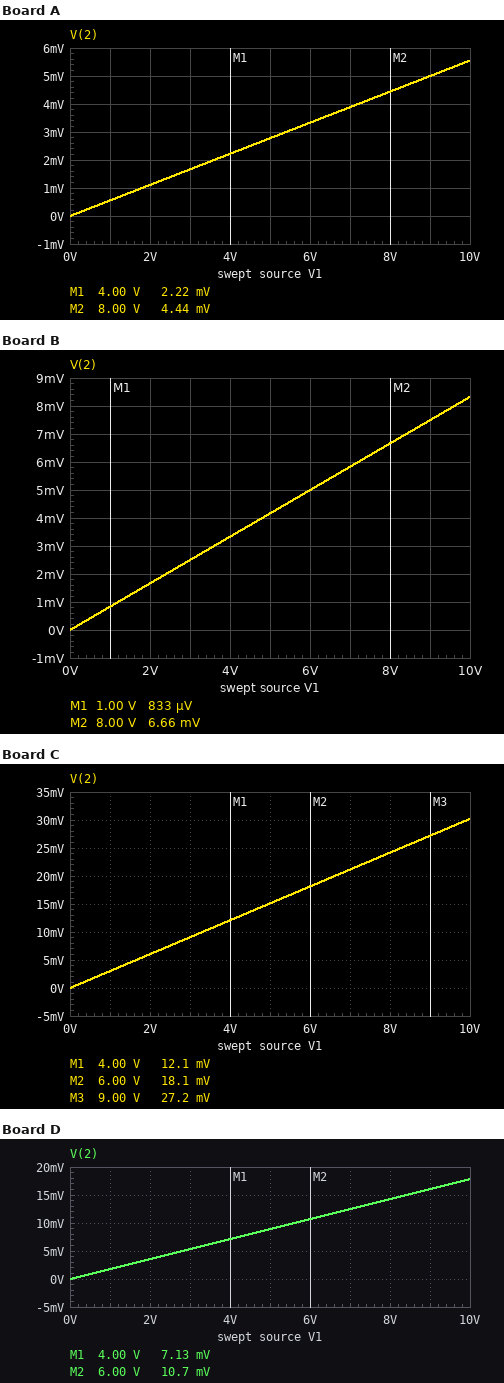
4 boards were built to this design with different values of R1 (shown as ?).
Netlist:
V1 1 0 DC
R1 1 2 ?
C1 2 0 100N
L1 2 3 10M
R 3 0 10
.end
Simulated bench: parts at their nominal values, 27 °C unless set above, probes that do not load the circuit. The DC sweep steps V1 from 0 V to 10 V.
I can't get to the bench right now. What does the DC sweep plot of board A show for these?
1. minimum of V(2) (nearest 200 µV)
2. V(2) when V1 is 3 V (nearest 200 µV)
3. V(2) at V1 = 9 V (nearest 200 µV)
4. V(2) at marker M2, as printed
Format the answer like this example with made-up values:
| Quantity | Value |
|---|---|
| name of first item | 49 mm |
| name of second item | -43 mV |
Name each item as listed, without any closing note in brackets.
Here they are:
| Quantity | Value |
|---|---|
| minimum of V(2) | 0 V |
| V(2) when V1 is 3 V | 1.6 mV |
| V(2) at V1 = 9 V | 5.0 mV |
| V(2) at marker M2, as printed | 4.44 mV |
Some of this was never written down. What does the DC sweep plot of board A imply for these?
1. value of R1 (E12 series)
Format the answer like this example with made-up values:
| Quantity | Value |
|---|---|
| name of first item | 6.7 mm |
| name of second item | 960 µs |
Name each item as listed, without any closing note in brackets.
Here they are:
| Quantity | Value |
|---|---|
| value of R1 | 18 kΩ |
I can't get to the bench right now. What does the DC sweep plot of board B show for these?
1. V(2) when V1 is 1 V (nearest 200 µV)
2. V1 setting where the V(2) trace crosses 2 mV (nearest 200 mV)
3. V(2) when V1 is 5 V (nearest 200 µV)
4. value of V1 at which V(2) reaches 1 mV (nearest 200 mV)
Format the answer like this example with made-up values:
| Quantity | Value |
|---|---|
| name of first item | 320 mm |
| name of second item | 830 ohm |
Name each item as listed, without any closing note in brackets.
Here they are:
| Quantity | Value |
|---|---|
| V(2) when V1 is 1 V | 800 µV |
| V1 setting where the V(2) trace crosses 2 mV | 2.4 V |
| V(2) when V1 is 5 V | 4.2 mV |
| value of V1 at which V(2) reaches 1 mV | 1.2 V |
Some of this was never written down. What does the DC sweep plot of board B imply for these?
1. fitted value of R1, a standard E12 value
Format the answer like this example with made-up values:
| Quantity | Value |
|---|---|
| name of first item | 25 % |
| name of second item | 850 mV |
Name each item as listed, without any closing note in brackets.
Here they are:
| Quantity | Value |
|---|---|
| fitted value of R1, a standard E12 value | 12 kΩ |
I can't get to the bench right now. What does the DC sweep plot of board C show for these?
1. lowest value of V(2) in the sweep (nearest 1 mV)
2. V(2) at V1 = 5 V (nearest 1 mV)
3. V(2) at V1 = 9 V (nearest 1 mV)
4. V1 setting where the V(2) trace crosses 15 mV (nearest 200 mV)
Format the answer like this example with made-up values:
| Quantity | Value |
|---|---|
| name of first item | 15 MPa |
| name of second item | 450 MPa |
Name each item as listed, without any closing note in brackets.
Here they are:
| Quantity | Value |
|---|---|
| lowest value of V(2) in the sweep | 0 V |
| V(2) at V1 = 5 V | 15 mV |
| V(2) at V1 = 9 V | 27 mV |
| V1 setting where the V(2) trace crosses 15 mV | 5.0 V |
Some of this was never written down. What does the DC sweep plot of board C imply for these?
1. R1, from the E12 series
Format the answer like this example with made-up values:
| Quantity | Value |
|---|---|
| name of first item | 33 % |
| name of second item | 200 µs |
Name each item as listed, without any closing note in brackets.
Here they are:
| Quantity | Value |
|---|---|
| R1, from the E12 series | 3.3 kΩ |
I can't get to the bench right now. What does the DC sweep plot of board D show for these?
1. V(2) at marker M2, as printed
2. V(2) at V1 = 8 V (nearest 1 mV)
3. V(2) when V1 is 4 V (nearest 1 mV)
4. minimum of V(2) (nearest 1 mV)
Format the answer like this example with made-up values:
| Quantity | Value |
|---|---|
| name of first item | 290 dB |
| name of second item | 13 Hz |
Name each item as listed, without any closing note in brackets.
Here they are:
| Quantity | Value |
|---|---|
| V(2) at marker M2, as printed | 10.7 mV |
| V(2) at V1 = 8 V | 14 mV |
| V(2) when V1 is 4 V | 7 mV |
| minimum of V(2) | 0 V |
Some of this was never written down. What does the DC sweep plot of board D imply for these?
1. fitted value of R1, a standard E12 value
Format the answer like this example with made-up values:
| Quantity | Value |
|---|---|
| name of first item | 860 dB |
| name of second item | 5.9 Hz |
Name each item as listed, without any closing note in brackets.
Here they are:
| Quantity | Value |
|---|---|
| fitted value of R1, a standard E12 value | 5.6 kΩ |
